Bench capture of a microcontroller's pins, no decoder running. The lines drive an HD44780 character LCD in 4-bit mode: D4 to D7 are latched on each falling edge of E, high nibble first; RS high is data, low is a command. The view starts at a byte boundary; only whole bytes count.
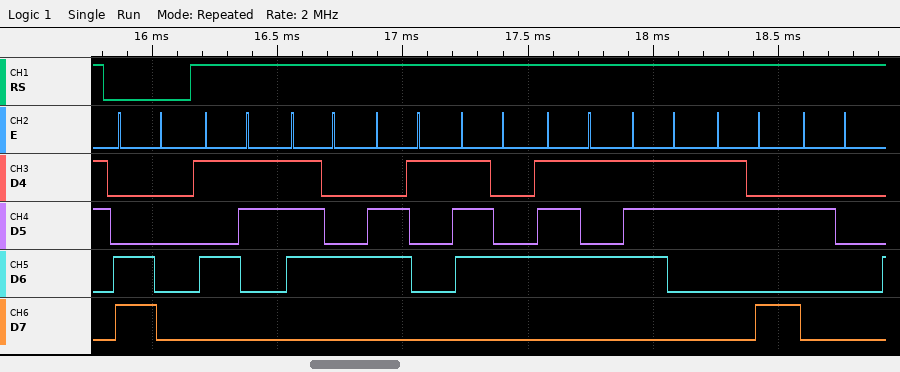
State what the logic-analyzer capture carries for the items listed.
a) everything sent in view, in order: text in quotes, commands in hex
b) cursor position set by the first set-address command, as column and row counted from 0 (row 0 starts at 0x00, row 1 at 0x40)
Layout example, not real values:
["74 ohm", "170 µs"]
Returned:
["0xC0 \"Status: \"", "column 0, row 1"]
